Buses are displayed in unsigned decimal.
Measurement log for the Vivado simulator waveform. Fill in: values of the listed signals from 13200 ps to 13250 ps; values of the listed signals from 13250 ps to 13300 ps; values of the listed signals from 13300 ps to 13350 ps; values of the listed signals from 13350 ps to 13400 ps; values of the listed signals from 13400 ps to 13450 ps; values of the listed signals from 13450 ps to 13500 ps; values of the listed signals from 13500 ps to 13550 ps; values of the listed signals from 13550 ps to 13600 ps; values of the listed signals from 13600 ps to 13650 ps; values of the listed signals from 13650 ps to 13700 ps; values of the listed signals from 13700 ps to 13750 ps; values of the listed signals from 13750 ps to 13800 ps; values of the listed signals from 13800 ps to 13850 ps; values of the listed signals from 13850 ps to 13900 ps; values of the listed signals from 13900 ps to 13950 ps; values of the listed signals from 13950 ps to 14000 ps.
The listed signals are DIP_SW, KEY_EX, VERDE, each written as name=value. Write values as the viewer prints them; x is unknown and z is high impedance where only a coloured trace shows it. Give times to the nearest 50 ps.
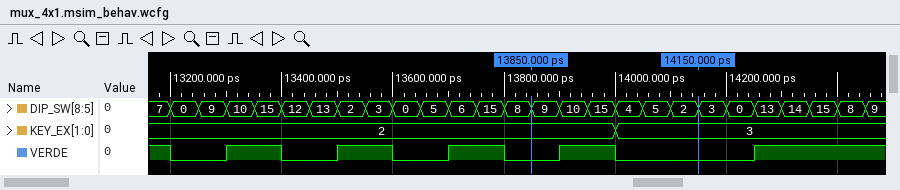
DIP_SW=0, KEY_EX=2, VERDE=0
DIP_SW=9, KEY_EX=2, VERDE=0
DIP_SW=10, KEY_EX=2, VERDE=1
DIP_SW=15, KEY_EX=2, VERDE=1
DIP_SW=12, KEY_EX=2, VERDE=0
DIP_SW=13, KEY_EX=2, VERDE=0
DIP_SW=2, KEY_EX=2, VERDE=1
DIP_SW=3, KEY_EX=2, VERDE=1
DIP_SW=0, KEY_EX=2, VERDE=0
DIP_SW=5, KEY_EX=2, VERDE=0
DIP_SW=6, KEY_EX=2, VERDE=1
DIP_SW=15, KEY_EX=2, VERDE=1
DIP_SW=8, KEY_EX=2, VERDE=0
DIP_SW=9, KEY_EX=2, VERDE=0
DIP_SW=10, KEY_EX=2, VERDE=1
DIP_SW=15, KEY_EX=2, VERDE=1
